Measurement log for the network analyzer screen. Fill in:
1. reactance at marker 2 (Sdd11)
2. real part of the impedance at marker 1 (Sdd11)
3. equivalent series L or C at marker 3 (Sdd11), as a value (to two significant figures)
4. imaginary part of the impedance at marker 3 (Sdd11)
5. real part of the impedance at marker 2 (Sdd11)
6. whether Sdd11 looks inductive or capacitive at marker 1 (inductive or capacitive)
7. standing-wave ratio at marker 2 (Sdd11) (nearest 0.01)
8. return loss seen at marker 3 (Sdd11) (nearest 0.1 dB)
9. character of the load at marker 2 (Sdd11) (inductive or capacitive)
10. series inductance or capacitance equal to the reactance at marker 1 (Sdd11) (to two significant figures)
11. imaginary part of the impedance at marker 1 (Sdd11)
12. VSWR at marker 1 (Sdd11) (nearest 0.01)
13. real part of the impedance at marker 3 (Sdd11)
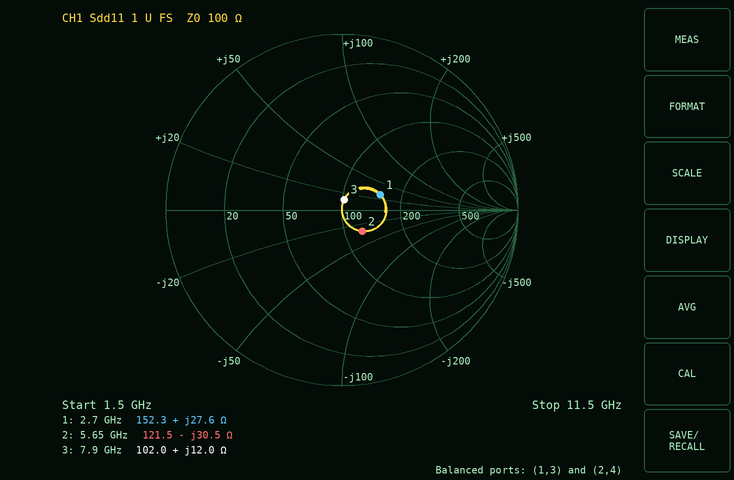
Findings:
-30.5 Ω
152.3 Ω
240 pH
+12.0 Ω
121.5 Ω
inductive
1.40
24.4 dB
capacitive
1.6 nH
+27.6 Ω
1.61
102.0 Ω
